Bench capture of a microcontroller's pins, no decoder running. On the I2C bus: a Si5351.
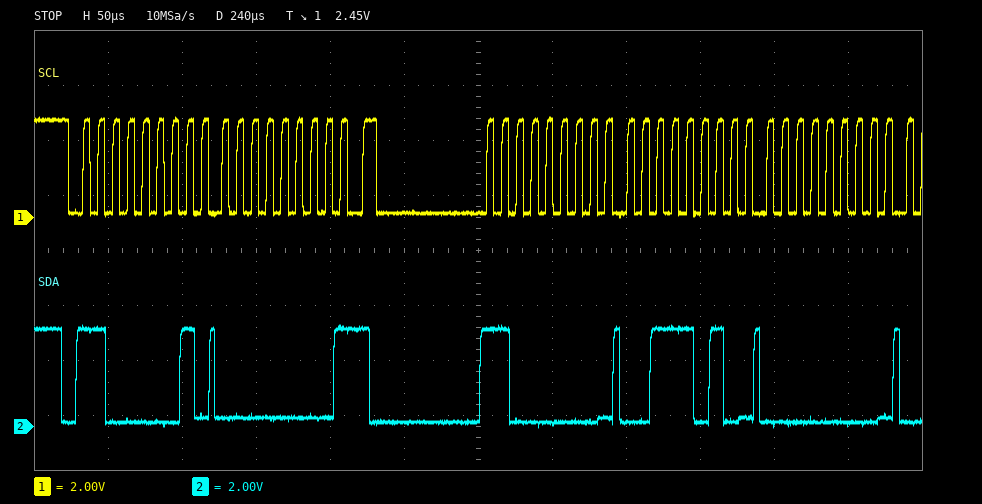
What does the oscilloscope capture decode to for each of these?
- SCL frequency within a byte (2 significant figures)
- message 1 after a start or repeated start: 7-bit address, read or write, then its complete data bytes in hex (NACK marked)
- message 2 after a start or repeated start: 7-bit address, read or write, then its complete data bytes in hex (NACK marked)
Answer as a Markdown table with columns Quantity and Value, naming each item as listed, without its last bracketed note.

| Quantity | Value |
|---|---|
| SCL frequency within a byte | 100 kHz |
| message 1 after a start or repeated start: 7-bit address, read or write, then its complete data bytes in hex | 0x60 read: 00 NACK |
| message 2 after a start or repeated start: 7-bit address, read or write, then its complete data bytes in hex | 0x60 write: 3A 00 |
